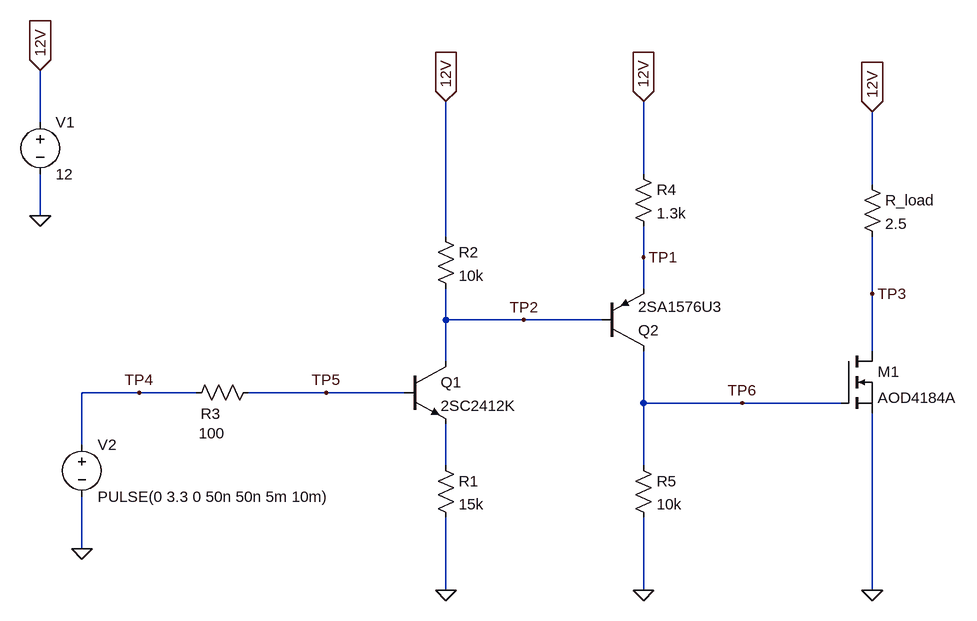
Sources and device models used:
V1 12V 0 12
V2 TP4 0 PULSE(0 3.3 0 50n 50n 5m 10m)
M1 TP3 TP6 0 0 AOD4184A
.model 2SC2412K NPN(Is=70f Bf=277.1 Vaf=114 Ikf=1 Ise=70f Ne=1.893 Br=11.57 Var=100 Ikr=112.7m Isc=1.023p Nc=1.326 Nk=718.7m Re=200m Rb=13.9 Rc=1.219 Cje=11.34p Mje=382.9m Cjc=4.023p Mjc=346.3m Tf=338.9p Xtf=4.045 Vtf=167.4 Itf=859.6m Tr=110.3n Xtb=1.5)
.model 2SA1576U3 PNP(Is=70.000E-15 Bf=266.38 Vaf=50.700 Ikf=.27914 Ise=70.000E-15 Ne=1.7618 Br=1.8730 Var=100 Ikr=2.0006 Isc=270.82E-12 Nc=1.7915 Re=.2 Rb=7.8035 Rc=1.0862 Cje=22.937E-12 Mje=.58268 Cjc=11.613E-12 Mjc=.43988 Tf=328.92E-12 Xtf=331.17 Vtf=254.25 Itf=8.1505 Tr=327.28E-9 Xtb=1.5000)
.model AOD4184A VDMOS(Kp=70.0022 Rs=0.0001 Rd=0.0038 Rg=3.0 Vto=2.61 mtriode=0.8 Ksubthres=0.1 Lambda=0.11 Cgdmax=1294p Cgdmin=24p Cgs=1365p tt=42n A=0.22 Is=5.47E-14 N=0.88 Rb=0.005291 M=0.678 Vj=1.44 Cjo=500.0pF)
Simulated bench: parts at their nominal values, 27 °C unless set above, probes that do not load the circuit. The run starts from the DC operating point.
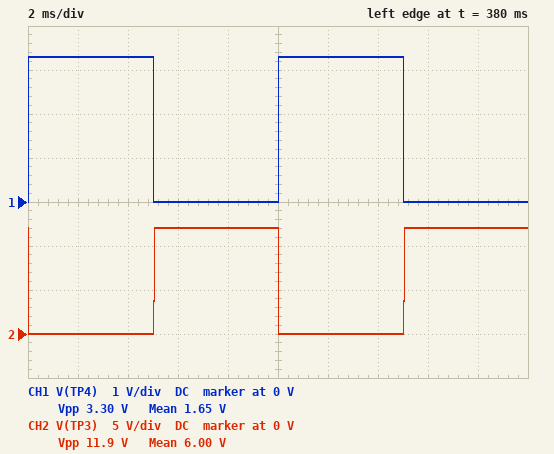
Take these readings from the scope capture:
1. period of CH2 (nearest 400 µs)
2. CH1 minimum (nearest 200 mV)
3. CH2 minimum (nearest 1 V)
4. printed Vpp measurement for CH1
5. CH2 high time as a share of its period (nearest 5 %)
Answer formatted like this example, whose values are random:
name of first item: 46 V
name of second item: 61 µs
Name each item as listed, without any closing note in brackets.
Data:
period of CH2: 10.0 ms
CH1 minimum: 0 V
CH2 minimum: 0 V
printed Vpp measurement for CH1: 3.30 V
CH2 high time as a share of its period: 50 %
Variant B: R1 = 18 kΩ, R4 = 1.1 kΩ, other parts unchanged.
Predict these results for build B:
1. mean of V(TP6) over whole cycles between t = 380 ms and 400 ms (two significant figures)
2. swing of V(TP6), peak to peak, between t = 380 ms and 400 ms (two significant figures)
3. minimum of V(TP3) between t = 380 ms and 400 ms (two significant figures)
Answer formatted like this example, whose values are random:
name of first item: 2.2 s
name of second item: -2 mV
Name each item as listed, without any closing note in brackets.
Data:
mean of V(TP6) over whole cycles between t = 380 ms and 400 ms: 4.0 V
swing of V(TP6), peak to peak, between t = 380 ms and 400 ms: 8.1 V
minimum of V(TP3) between t = 380 ms and 400 ms: 34 mV
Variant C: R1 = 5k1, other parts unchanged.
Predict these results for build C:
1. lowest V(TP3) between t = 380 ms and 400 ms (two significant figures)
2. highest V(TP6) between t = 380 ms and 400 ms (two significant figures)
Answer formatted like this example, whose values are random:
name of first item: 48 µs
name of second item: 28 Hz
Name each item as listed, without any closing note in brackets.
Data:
lowest V(TP3) between t = 380 ms and 400 ms: 30 mV
highest V(TP6) between t = 380 ms and 400 ms: 10 V
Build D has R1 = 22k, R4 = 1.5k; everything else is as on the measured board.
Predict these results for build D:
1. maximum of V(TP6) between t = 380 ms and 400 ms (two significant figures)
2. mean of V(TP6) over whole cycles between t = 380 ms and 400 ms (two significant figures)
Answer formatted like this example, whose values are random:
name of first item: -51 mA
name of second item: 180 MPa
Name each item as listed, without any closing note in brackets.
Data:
maximum of V(TP6) between t = 380 ms and 400 ms: 4.3 V
mean of V(TP6) over whole cycles between t = 380 ms and 400 ms: 2.2 V
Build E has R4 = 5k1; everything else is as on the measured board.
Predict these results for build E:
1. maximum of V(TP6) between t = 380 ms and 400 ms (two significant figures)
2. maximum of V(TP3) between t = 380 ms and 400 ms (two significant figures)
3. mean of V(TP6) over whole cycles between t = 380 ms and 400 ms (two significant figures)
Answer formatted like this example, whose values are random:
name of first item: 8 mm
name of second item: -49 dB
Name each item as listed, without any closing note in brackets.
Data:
maximum of V(TP6) between t = 380 ms and 400 ms: 2.4 V
maximum of V(TP3) between t = 380 ms and 400 ms: 12 V
mean of V(TP6) over whole cycles between t = 380 ms and 400 ms: 1.2 V
